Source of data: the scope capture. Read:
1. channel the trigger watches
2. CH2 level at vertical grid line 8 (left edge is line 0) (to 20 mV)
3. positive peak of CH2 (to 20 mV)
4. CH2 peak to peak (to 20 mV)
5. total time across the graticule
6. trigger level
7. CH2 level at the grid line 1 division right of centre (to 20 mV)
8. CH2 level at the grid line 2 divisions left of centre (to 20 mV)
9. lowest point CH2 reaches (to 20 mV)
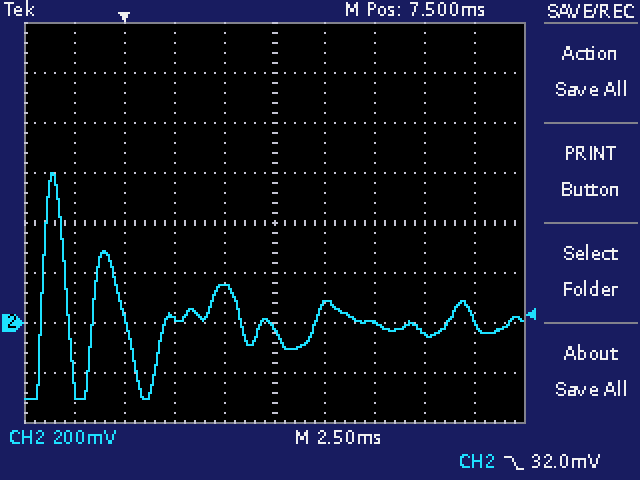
CH2
-40 mV
600 mV
900 mV
25 ms
32.0 mV
80 mV
20 mV
-300 mV
